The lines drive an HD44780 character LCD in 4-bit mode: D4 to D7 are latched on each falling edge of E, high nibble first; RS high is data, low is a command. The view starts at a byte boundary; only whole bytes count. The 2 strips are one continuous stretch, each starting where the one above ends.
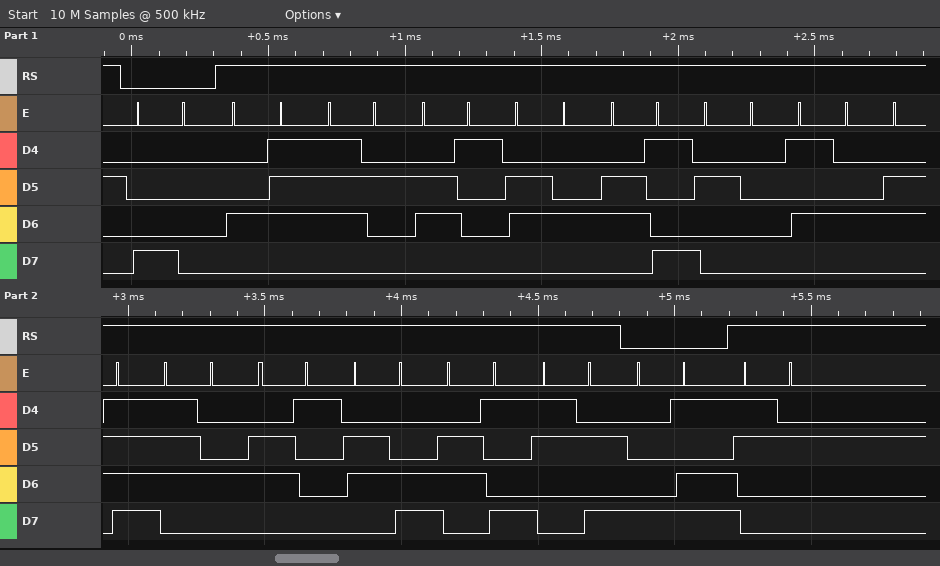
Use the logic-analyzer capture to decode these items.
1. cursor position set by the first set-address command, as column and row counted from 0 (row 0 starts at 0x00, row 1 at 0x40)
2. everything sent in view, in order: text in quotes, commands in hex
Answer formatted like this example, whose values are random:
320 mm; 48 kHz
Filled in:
column 0, row 0; 0x80 "Gradi Totali:" 0x8D "2"
